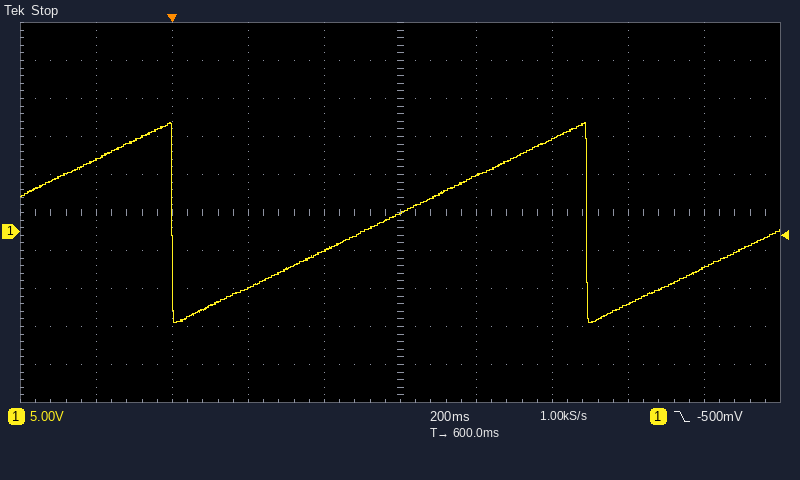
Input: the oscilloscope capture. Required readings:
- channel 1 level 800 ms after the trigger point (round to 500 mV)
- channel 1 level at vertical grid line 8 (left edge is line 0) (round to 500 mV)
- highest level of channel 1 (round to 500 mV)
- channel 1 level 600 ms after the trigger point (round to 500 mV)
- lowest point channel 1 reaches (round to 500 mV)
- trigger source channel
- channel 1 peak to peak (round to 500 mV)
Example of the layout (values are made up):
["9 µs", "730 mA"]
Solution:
["7.5 V", "-9.5 V", "14.5 V", "2.5 V", "-12.0 V", "channel 1", "26.5 V"]
